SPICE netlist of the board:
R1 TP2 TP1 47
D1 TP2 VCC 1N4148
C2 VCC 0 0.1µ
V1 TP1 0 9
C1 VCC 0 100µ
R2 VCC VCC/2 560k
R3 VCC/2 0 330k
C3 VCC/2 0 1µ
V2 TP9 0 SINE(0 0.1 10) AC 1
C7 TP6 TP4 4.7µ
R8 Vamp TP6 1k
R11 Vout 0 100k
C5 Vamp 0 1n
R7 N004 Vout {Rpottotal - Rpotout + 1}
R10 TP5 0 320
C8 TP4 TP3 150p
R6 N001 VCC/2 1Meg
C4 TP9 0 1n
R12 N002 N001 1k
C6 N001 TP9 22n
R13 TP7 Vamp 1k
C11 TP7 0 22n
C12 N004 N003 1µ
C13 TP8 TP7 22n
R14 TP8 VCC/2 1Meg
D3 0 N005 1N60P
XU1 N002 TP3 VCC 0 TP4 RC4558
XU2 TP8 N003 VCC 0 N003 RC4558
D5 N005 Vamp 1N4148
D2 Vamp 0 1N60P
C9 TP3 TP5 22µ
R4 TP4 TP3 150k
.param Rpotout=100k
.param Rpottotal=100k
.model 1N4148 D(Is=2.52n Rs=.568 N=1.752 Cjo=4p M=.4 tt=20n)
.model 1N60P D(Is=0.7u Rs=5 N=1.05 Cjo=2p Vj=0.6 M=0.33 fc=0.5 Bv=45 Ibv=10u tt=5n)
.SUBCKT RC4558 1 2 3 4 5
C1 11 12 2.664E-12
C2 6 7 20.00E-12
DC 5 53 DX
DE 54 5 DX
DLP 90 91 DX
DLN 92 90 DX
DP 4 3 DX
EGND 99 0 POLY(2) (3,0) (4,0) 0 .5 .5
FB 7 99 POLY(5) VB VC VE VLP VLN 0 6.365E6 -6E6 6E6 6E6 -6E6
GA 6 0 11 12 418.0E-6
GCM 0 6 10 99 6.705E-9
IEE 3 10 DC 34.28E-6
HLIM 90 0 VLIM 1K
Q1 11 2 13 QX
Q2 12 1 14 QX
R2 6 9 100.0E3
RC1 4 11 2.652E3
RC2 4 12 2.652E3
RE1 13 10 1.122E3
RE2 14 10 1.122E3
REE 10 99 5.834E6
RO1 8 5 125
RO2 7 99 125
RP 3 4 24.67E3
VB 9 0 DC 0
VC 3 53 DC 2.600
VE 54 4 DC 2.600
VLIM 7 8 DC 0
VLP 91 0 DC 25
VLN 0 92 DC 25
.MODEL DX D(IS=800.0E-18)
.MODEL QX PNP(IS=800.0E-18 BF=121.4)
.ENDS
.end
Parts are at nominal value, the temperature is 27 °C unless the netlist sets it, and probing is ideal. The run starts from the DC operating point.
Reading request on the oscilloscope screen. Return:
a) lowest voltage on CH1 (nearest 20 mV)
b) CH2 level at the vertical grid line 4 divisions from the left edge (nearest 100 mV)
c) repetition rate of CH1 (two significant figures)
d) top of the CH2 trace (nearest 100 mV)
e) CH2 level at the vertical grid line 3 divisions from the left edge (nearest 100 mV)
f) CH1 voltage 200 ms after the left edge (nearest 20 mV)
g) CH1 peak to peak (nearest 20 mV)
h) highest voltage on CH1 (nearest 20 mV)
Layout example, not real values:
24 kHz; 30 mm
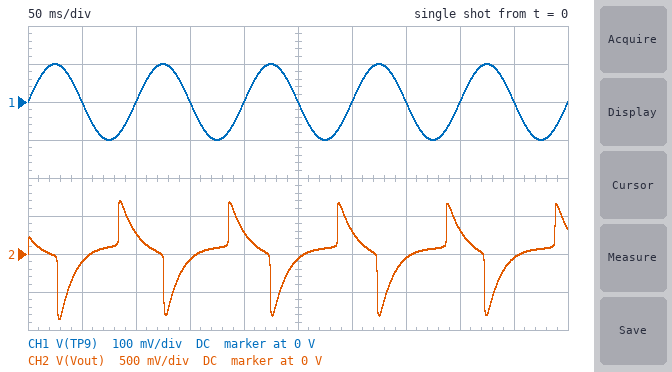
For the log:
-100 mV; 300 mV; 10 Hz; 700 mV; -100 mV; 0 V; 200 mV; 100 mV
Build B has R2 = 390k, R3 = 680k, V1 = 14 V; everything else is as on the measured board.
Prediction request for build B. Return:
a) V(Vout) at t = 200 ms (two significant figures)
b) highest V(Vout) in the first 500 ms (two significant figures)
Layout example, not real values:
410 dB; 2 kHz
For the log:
65 mV; 770 mV
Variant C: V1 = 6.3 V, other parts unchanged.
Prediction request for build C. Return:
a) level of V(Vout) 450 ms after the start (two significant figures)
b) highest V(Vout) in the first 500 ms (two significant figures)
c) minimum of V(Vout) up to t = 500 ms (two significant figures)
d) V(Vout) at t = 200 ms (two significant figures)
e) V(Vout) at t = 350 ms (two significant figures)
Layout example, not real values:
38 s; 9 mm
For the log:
-110 mV; 650 mV; -430 mV; 260 mV; -120 mV
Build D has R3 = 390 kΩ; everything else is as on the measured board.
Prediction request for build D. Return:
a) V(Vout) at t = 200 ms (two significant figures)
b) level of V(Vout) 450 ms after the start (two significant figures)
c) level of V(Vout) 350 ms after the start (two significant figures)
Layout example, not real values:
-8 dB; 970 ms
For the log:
250 mV; -88 mV; -91 mV
